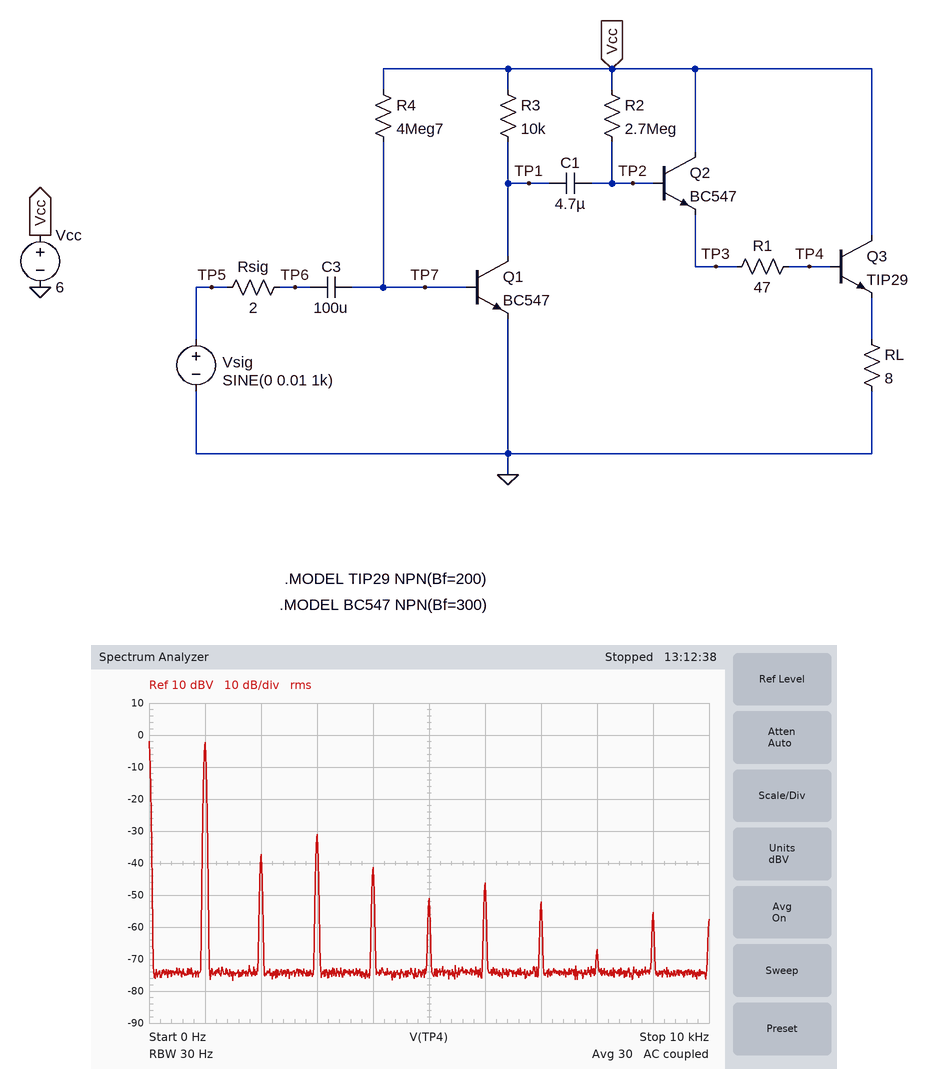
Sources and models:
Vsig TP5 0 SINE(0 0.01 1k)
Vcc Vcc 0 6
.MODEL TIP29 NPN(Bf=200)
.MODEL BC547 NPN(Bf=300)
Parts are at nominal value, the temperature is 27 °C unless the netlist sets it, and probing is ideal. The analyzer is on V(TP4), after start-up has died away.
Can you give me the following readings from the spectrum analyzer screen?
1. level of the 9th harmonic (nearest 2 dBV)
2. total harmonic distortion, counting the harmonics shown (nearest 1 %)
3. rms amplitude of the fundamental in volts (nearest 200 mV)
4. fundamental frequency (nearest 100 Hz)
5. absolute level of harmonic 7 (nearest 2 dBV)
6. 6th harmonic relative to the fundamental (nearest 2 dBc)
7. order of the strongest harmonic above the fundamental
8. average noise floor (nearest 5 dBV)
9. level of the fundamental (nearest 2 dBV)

-56 dBV
4 %
800 mV
1.0 kHz
-52 dBV
-44 dBc
3
-75 dBV
-2 dBV
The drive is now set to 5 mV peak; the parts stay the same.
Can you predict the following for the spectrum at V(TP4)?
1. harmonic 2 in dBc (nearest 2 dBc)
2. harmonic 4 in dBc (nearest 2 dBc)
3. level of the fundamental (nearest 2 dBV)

-28 dBc
-54 dBc
-8 dBV
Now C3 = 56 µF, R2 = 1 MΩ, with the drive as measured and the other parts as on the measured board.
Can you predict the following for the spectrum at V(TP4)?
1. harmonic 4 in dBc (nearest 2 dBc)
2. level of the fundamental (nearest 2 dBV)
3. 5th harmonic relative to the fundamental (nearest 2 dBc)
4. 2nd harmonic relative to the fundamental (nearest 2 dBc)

-52 dBc
-2 dBV
-56 dBc
-22 dBc
